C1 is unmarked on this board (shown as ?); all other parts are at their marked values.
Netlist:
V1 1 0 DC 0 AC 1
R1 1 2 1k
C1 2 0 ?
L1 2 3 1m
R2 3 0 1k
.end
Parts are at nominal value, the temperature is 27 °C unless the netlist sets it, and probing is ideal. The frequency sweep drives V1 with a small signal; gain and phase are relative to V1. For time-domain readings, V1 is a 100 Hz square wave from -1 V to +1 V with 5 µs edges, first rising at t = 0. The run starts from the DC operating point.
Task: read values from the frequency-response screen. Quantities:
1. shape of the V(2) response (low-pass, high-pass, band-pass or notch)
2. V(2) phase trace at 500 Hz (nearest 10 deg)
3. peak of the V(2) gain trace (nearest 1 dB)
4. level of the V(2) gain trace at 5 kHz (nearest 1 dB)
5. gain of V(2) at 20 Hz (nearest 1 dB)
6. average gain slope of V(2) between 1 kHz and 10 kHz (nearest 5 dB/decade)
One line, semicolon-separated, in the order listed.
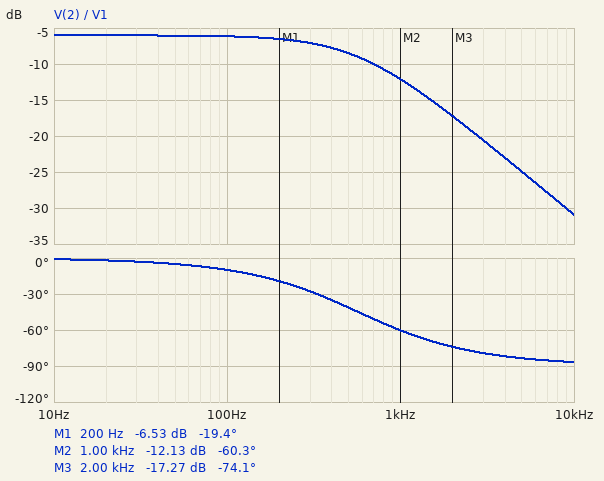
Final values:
low-pass; -40 deg; -6 dB; -25 dB; -6 dB; -20 dB/decade
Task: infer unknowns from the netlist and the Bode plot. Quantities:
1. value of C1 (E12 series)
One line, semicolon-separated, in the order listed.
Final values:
560 nF
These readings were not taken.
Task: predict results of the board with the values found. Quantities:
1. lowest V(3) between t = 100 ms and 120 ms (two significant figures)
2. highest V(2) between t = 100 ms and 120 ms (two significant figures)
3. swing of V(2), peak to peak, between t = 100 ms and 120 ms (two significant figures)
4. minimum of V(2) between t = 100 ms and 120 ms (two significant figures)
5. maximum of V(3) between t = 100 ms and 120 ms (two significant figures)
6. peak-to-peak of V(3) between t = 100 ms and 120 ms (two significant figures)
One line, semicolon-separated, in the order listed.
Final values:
-500 mV; 500 mV; 1.0 V; -500 mV; 500 mV; 1.0 V
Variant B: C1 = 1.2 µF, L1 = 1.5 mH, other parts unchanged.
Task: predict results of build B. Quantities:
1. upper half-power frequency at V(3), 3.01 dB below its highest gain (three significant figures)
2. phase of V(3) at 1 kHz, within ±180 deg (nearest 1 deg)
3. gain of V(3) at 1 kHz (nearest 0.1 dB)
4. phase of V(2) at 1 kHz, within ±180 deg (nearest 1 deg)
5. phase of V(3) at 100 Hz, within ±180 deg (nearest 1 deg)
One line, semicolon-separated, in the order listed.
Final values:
266 Hz; -76 deg; -17.8 dB; -75 deg; -21 deg
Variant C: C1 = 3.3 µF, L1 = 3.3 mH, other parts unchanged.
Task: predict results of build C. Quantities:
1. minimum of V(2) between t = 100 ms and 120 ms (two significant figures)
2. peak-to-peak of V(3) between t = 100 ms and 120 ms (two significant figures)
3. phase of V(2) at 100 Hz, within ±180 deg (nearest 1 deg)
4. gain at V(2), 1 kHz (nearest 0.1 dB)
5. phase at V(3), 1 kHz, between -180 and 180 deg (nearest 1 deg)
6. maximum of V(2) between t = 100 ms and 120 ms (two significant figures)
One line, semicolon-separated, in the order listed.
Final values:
-450 mV; 910 mV; -46 deg; -26.4 dB; -86 deg; 450 mV
